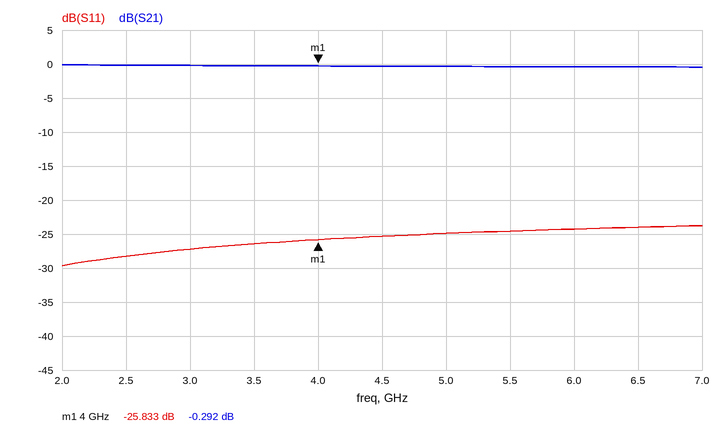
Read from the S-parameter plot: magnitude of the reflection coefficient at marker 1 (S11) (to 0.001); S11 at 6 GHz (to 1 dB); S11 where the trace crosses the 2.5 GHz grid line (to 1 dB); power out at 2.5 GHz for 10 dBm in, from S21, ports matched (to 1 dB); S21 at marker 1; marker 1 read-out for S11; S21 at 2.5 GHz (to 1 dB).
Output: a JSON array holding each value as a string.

["0.051", "-24 dB", "-28 dB", "10 dBm", "-0.292 dB", "-25.833 dB", "0 dB"]
